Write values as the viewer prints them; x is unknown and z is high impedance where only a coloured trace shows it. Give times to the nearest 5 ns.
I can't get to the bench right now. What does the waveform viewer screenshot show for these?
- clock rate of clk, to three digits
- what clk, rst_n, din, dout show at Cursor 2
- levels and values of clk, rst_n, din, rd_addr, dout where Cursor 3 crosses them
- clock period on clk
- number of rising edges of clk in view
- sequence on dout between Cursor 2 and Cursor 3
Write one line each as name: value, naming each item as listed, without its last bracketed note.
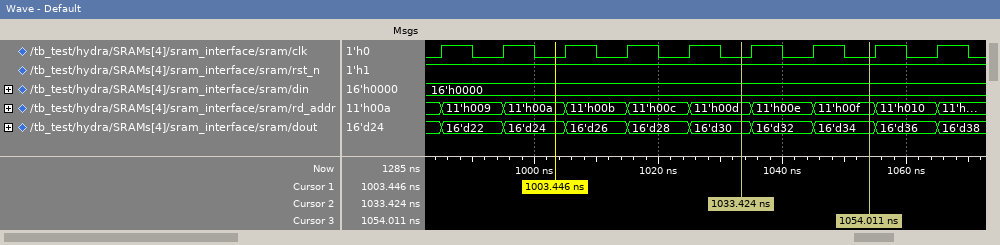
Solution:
clock rate of clk, to three digits: 100 MHz
what clk, rst_n, din, dout show at Cursor 2: clk=0, rst_n=1, din=16'h0000, dout=16'd30
levels and values of clk, rst_n, din, rd_addr, dout where Cursor 3 crosses them: clk=0, rst_n=1, din=16'h0000, rd_addr=11'h00f, dout=16'd34
clock period on clk: 10 ns
number of rising edges of clk in view: 9
sequence on dout between Cursor 2 and Cursor 3: 16'd30, 16'd32, 16'd34
